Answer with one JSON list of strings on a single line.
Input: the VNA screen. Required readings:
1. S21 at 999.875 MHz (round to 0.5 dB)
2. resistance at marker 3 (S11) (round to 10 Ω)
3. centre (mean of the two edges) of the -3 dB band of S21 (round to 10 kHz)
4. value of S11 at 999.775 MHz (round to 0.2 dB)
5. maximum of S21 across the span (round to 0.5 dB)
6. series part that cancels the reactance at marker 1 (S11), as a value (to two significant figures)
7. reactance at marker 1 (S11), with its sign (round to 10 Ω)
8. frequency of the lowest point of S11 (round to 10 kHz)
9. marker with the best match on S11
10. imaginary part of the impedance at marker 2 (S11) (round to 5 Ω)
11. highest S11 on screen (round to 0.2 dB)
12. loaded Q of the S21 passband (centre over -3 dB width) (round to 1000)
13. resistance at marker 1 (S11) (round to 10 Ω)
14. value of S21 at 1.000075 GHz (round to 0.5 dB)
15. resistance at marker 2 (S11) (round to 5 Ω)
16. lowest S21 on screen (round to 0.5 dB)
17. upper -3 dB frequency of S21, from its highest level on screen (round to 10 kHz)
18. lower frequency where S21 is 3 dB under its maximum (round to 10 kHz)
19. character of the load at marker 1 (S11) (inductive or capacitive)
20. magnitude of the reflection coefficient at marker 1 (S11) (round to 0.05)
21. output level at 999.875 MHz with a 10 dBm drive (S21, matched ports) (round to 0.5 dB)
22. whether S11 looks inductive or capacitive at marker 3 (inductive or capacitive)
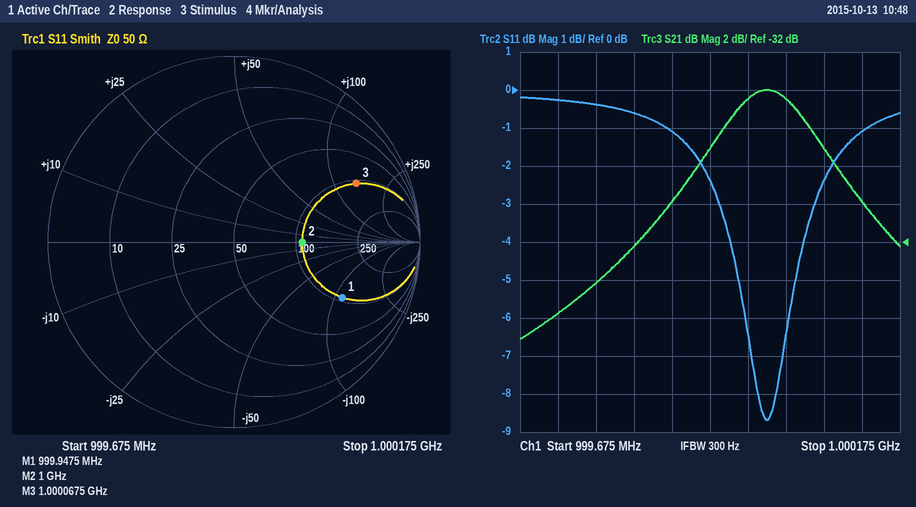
["-30.0 dB", "110 Ω", "1.00000 GHz", "-0.4 dB", "-24.0 dB", "18 nH", "-110 Ω", "1.00000 GHz", "marker 2", "0 Ω", "-0.2 dB", "7000", "110 Ω", "-27.0 dB", "110 Ω", "-37.0 dB", "1.00007 GHz", "999.93 MHz", "capacitive", "0.65", "-20.0 dBm", "inductive"]
